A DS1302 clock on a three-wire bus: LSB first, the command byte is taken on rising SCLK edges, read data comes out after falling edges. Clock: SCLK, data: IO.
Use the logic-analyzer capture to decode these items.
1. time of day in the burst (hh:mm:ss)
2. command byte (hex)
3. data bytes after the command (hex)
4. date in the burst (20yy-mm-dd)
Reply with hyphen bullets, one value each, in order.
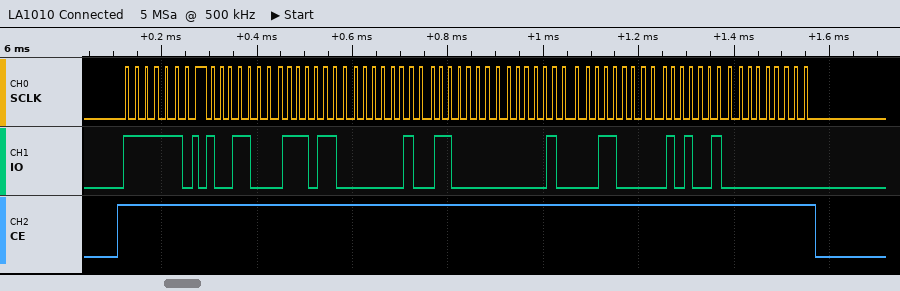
- 20:37:19
- 0xBF
- 19 37 20 03 10 06 25 00
- 2025-10-03
